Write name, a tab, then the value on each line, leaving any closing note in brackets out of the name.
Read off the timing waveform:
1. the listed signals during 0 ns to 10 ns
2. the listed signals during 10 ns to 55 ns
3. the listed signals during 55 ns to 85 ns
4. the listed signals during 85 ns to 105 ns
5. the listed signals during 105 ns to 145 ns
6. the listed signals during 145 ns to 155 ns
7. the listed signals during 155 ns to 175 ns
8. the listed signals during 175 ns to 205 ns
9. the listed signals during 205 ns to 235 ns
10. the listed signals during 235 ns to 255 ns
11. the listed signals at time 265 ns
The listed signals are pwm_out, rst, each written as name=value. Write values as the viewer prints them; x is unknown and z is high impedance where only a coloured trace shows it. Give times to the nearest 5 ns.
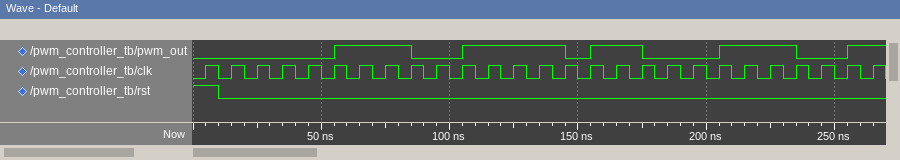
the listed signals during 0 ns to 10 ns	pwm_out=0, rst=1
the listed signals during 10 ns to 55 ns	pwm_out=0, rst=0
the listed signals during 55 ns to 85 ns	pwm_out=1, rst=0
the listed signals during 85 ns to 105 ns	pwm_out=0, rst=0
the listed signals during 105 ns to 145 ns	pwm_out=1, rst=0
the listed signals during 145 ns to 155 ns	pwm_out=0, rst=0
the listed signals during 155 ns to 175 ns	pwm_out=1, rst=0
the listed signals during 175 ns to 205 ns	pwm_out=0, rst=0
the listed signals during 205 ns to 235 ns	pwm_out=1, rst=0
the listed signals during 235 ns to 255 ns	pwm_out=0, rst=0
the listed signals at time 265 ns	pwm_out=1, rst=0
